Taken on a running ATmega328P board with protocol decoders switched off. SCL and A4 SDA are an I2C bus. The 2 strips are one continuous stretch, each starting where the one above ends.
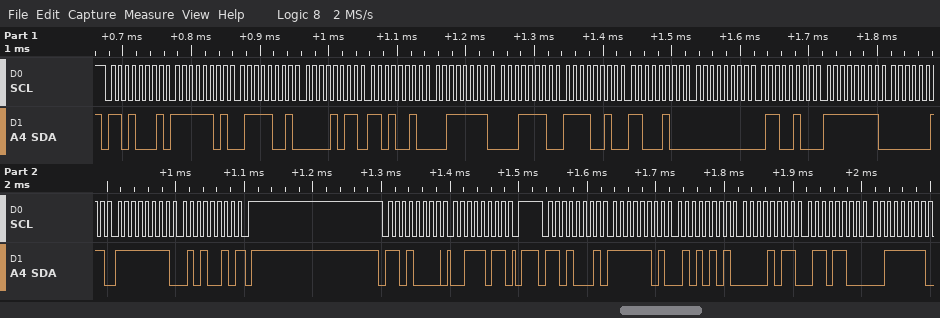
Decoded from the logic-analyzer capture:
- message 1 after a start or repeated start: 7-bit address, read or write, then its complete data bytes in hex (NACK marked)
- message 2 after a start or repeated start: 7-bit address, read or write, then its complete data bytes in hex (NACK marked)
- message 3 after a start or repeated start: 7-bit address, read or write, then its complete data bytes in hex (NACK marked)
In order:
0x68 read: FD 79 0B D2 3F 1E F2 C4 00 64 FF 03 FF 52 NACK
0x68 write: 3B
0x68 read: FD 55 0B 6C 3F
